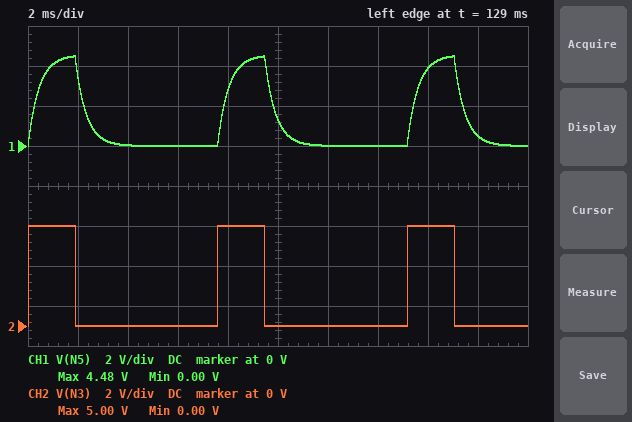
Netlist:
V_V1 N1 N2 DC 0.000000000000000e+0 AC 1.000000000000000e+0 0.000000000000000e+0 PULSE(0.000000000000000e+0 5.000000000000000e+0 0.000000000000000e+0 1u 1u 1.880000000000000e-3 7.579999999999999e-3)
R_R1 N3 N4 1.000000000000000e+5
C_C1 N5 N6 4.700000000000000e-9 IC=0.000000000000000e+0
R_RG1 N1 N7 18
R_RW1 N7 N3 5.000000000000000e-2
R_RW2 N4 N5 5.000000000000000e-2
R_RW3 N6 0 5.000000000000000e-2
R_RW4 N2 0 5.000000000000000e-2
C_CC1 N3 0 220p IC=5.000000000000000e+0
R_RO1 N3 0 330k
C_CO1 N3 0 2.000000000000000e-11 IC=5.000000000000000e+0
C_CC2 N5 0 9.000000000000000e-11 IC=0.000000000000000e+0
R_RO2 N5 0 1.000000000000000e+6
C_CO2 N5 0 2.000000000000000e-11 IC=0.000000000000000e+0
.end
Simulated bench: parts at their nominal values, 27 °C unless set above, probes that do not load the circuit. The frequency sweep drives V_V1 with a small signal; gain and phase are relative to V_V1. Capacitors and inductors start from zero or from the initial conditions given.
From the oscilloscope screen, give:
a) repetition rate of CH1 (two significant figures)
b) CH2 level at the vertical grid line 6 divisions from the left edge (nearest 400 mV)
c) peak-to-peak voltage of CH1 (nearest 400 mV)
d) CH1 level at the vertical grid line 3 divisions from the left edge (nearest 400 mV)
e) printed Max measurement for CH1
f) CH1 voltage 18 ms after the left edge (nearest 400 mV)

130 Hz
0 V
4.4 V
0 V
4.48 V
400 mV
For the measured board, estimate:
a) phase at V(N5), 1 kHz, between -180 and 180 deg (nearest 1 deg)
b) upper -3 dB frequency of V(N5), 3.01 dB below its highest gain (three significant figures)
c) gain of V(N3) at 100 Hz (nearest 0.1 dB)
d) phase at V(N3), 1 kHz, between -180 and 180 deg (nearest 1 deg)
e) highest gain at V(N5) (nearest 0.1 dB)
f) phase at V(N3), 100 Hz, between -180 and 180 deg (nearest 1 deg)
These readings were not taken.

-70 deg
364 Hz
0 dB
0 deg
-0.8 dB
0 deg
